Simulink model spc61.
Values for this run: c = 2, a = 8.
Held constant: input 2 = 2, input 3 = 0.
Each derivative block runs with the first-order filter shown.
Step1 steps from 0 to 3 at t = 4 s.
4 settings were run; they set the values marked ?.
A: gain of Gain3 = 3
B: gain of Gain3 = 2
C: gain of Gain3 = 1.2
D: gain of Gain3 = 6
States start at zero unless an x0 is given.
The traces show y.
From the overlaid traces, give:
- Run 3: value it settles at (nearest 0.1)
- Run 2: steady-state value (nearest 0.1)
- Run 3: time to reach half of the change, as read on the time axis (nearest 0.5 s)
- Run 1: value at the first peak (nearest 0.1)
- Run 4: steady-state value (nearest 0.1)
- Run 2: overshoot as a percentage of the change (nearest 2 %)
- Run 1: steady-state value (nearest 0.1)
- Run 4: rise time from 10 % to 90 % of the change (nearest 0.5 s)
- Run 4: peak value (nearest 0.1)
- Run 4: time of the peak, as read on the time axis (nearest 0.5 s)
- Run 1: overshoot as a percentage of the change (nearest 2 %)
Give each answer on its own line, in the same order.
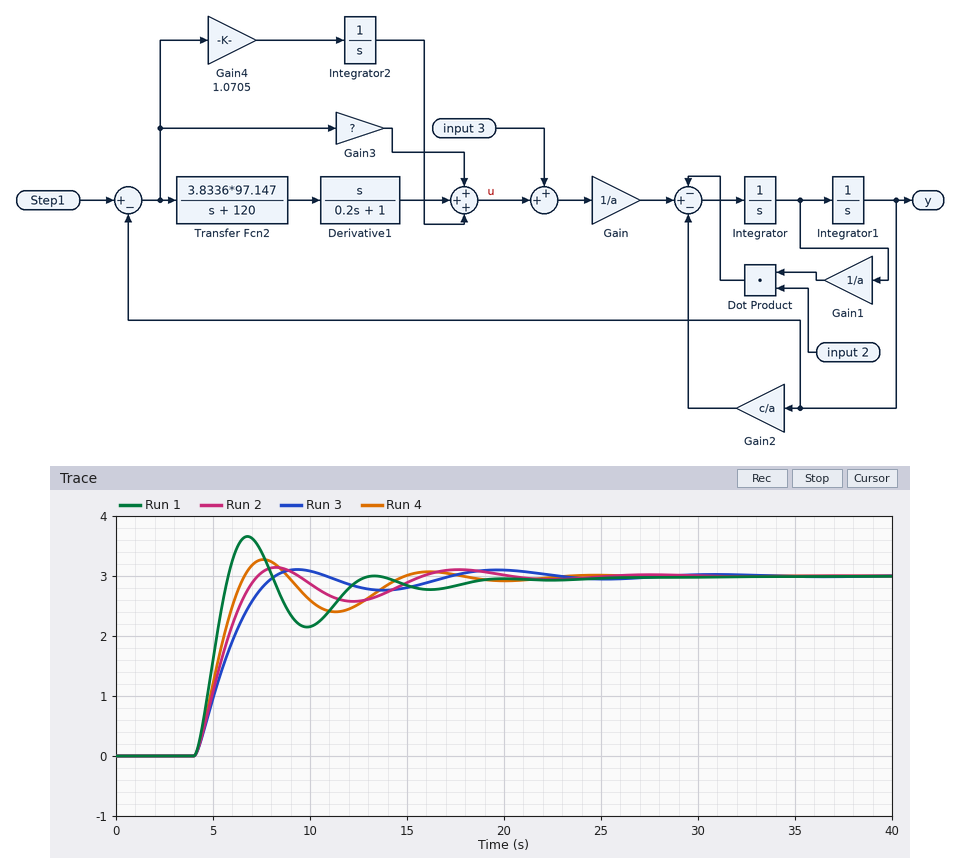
3.0
3.0
5.5 s
3.7
3.0
4 %
3.0
2.0 s
3.3
7.5 s
22 %
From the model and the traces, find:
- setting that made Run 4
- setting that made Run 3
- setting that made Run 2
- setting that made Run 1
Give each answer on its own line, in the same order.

A
C
B
D
